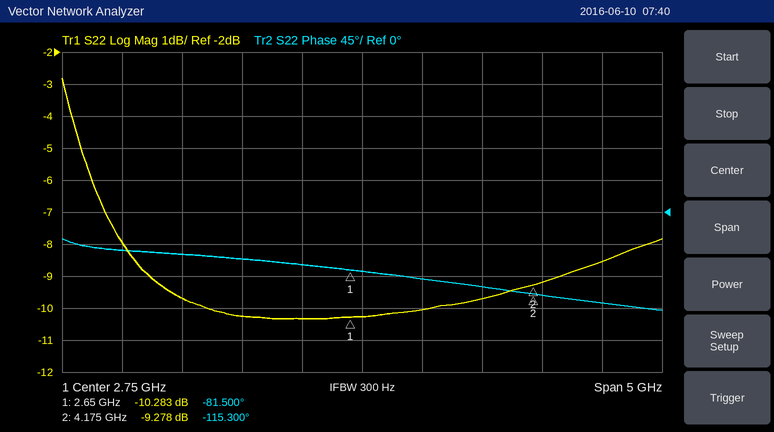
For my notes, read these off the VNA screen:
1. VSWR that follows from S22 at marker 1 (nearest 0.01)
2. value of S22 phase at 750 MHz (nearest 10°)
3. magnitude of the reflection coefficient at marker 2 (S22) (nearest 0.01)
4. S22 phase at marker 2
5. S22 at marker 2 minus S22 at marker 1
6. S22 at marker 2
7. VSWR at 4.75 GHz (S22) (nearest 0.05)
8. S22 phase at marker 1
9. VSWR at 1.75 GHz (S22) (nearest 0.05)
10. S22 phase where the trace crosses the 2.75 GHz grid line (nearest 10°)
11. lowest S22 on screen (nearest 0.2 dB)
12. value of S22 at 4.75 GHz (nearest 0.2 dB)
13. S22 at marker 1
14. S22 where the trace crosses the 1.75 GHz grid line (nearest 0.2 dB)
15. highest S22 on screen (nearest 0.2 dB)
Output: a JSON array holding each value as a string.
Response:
["1.88", "-50°", "0.34", "-115.300°", "1.005 dB", "-9.278 dB", "2.20", "-81.500°", "1.90", "-80°", "-10.4 dB", "-8.6 dB", "-10.283 dB", "-10.2 dB", "-2.8 dB"]
